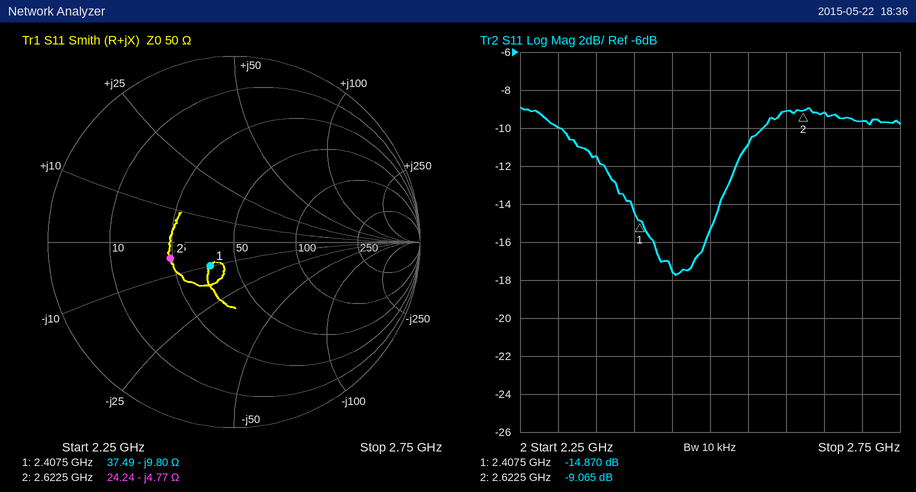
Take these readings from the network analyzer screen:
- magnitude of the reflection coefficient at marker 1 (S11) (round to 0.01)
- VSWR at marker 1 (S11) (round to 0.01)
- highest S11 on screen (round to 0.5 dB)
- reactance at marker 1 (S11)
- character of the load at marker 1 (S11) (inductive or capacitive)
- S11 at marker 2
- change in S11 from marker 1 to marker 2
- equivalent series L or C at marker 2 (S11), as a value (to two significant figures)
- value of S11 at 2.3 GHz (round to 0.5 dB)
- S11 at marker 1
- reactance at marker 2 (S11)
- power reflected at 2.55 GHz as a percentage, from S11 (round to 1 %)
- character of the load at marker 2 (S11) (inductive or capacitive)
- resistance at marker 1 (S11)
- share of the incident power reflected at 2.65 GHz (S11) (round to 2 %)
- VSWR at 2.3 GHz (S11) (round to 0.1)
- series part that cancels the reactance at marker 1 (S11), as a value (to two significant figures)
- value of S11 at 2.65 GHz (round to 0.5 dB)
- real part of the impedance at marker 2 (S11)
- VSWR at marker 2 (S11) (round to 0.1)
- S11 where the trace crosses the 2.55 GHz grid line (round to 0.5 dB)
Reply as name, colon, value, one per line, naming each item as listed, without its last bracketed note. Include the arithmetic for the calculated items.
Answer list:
magnitude of the reflection coefficient at marker 1 (S11): 0.18
VSWR at marker 1 (S11): (1 + 0.1805)/(1 − 0.1805) ≈ 1.44
highest S11 on screen: -9.0 dB
reactance at marker 1: -9.80 Ω
character of the load at marker 1 (S11): capacitive
S11 at marker 2: -9.065 dB
change in S11 from marker 1 to marker 2: -9.065 − (-14.87) = 5.805 dB
equivalent series L or C at marker 2 (S11), as a value: C = 1/(2π × 2.6225 GHz × 4.77 Ω) ≈ 13 pF
value of S11 at 2.3 GHz: -10.0 dB
S11 at marker 1: -14.870 dB
reactance at marker 2: -4.77 Ω
power reflected at 2.55 GHz as a percentage, from S11: 10^(-11/10) ≈ 8 %
character of the load at marker 2 (S11): capacitive
resistance at marker 1: 37.49 Ω
share of the incident power reflected at 2.65 GHz (S11): 10^(-9/10) ≈ 12.6 %, so 12 % to the nearest 2 %
VSWR at 2.3 GHz (S11): |Γ| = 10^(-10/20) = 0.3162; VSWR = (1 + 0.3162)/(1 − 0.3162) ≈ 1.9
series part that cancels the reactance at marker 1 (S11), as a value: L = 9.8 Ω/(2π × 2.4075 GHz) ≈ 648 pH, so 650 pH to two significant figures
value of S11 at 2.65 GHz: -9.0 dB
real part of the impedance at marker 2: 24.24 Ω
VSWR at marker 2 (S11): 2.1
S11 where the trace crosses the 2.55 GHz grid line: -11.0 dB
